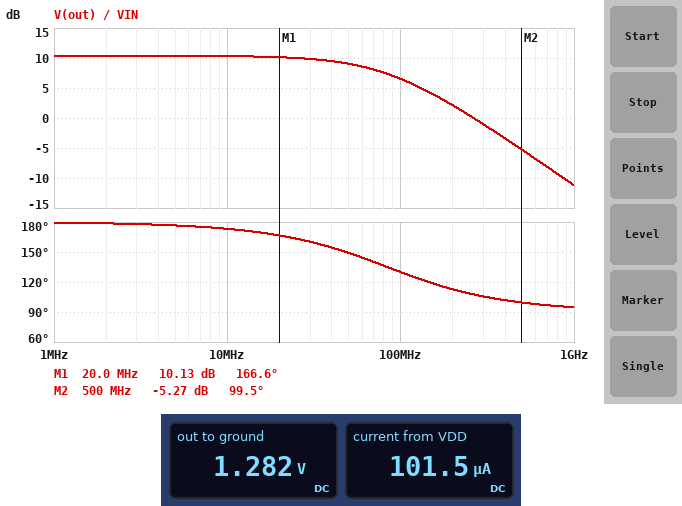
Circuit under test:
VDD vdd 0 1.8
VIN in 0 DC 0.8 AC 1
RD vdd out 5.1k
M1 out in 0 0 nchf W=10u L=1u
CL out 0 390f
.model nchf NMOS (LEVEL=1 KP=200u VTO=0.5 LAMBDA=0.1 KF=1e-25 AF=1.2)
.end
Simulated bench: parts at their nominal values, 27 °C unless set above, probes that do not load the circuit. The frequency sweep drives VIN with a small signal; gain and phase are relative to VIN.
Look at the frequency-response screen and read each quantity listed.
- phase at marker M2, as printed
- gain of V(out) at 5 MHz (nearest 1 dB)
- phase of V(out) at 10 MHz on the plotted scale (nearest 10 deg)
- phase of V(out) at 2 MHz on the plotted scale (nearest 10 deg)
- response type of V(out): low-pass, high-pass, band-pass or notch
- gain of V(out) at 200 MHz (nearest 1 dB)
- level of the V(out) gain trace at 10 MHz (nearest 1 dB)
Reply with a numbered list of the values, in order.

1. 99.5 deg
2. 10 dB
3. 170 deg
4. 180 deg
5. low-pass
6. 2 dB
7. 10 dB
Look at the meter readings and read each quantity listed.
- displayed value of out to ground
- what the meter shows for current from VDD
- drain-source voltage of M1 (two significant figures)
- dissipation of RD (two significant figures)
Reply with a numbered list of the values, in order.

1. 1.282 V
2. 101.5 µA
3. 1.3 V
4. 53 µW
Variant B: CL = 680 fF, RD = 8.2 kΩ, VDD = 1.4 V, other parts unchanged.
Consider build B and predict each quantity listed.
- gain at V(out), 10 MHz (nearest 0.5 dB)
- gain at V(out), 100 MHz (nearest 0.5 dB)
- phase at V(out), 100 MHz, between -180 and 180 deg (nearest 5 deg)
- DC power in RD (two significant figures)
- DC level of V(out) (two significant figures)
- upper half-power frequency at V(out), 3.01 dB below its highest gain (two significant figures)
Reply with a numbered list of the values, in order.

1. 13.5 dB
2. 3.0 dB
3. 105 deg
4. 75 µW
5. 620 mV
6. 31 MHz
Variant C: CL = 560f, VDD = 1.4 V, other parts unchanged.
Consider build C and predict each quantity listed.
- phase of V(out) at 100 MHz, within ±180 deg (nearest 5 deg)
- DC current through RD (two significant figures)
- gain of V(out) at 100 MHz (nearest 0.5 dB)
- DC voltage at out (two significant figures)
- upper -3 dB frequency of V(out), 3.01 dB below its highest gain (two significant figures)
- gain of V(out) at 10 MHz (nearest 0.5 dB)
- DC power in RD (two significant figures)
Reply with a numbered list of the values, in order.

1. 120 deg
2. 98 µA
3. 4.0 dB
4. 900 mV
5. 58 MHz
6. 10.0 dB
7. 49 µW
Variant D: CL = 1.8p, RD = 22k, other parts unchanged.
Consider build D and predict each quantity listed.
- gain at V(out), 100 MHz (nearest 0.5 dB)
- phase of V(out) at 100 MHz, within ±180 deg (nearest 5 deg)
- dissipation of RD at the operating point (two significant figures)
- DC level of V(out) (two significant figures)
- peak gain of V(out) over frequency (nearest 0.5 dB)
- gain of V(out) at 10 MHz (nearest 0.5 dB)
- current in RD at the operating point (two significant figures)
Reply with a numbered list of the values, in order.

1. -10.5 dB
2. 105 deg
3. 120 µW
4. 170 mV
5. 0.5 dB
6. 0 dB
7. 74 µA
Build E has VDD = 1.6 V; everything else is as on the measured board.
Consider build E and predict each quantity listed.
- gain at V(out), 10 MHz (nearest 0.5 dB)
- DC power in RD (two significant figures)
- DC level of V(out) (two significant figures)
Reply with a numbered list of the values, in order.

1. 10.0 dB
2. 51 µW
3. 1.1 V
